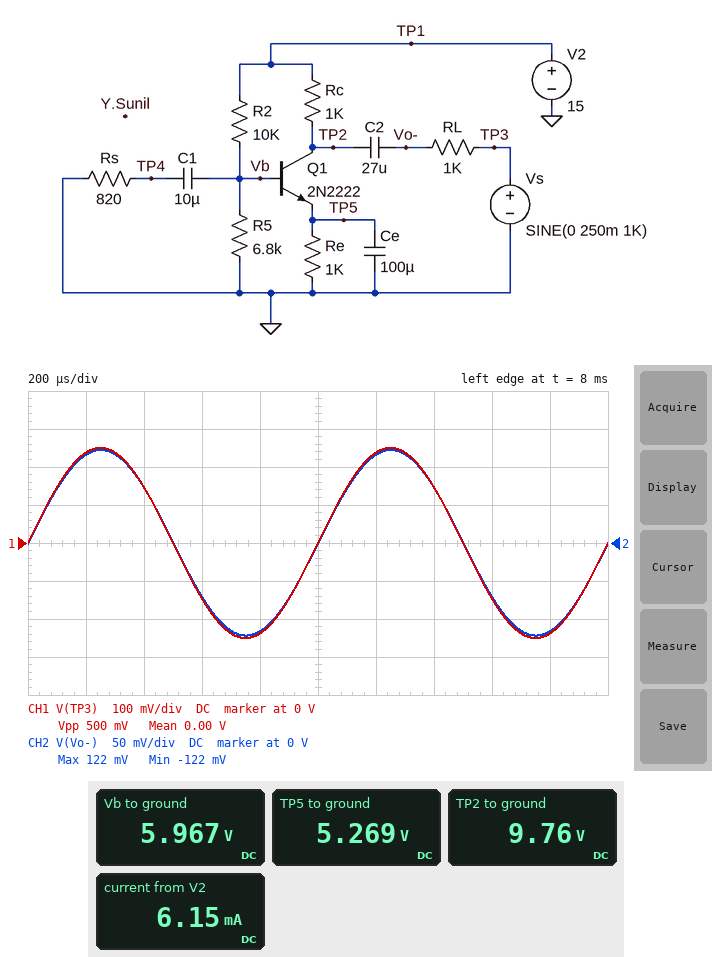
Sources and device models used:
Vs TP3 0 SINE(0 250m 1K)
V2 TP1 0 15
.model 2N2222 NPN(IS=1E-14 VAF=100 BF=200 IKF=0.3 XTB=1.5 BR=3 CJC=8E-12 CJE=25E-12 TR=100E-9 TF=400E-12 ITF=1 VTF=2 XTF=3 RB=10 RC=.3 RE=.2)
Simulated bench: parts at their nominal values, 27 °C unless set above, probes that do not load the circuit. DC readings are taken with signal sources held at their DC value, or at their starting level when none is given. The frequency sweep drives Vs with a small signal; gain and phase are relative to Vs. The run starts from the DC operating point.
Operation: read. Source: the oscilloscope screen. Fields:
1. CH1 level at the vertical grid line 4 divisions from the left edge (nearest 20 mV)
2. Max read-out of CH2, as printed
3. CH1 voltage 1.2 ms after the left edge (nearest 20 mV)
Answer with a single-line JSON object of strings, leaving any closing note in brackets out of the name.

{"CH1 level at the vertical grid line 4 divisions from the left edge": "-240 mV", "Max read-out of CH2, as printed": "122 mV", "CH1 voltage 1.2 ms after the left edge": "240 mV"}
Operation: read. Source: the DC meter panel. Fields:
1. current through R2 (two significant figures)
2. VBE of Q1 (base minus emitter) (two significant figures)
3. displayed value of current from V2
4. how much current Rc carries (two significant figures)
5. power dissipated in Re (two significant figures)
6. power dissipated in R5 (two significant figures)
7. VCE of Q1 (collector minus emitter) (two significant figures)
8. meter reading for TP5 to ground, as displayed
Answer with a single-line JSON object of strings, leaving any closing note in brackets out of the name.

{"current through R2": "900 µA", "VBE of Q1 (base minus emitter)": "700 mV", "displayed value of current from V2": "6.15 mA", "how much current Rc carries": "5.2 mA", "power dissipated in Re": "28 mW", "power dissipated in R5": "5.2 mW", "VCE of Q1 (collector minus emitter)": "4.5 V", "meter reading for TP5 to ground, as displayed": "5.269 V"}
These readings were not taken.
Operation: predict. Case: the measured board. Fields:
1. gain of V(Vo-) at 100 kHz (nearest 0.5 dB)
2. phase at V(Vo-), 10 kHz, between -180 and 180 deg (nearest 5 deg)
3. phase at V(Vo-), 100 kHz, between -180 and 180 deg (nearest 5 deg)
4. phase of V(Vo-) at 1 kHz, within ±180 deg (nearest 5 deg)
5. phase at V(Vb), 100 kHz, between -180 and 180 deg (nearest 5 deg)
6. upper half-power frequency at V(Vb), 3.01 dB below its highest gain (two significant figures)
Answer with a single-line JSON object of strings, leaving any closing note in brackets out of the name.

{"gain of V(Vo-) at 100 kHz": "-6.5 dB", "phase at V(Vo-), 10 kHz, between -180 and 180 deg": "0 deg", "phase at V(Vo-), 100 kHz, between -180 and 180 deg": "-5 deg", "phase of V(Vo-) at 1 kHz, within ±180 deg": "0 deg", "phase at V(Vb), 100 kHz, between -180 and 180 deg": "80 deg", "upper half-power frequency at V(Vb), 3.01 dB below its highest gain": "340 MHz"}
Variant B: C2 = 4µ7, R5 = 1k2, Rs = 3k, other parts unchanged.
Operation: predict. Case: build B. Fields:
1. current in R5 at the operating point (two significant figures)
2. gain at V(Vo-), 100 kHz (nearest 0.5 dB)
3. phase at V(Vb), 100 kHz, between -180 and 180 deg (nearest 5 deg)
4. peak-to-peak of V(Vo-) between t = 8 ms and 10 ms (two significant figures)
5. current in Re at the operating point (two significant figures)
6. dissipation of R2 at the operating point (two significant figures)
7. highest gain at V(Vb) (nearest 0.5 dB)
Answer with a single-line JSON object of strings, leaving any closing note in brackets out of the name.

{"current in R5 at the operating point": "1.3 mA", "gain at V(Vo-), 100 kHz": "-6.0 dB", "phase at V(Vb), 100 kHz, between -180 and 180 deg": "85 deg", "peak-to-peak of V(Vo-) between t = 8 ms and 10 ms": "250 mV", "current in Re at the operating point": "950 µA", "dissipation of R2 at the operating point": "18 mW", "highest gain at V(Vb)": "-37.5 dB"}
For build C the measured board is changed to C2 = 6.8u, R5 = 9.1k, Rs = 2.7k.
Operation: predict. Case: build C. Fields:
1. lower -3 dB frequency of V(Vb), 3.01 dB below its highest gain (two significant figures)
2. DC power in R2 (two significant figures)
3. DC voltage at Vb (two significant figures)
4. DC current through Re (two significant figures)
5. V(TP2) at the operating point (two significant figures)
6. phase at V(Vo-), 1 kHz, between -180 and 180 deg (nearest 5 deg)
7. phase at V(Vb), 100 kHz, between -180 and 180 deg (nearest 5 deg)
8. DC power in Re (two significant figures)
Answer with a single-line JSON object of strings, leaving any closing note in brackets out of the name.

{"lower -3 dB frequency of V(Vb), 3.01 dB below its highest gain": "380 kHz", "DC power in R2": "6.4 mW", "DC voltage at Vb": "7.0 V", "DC current through Re": "6.3 mA", "V(TP2) at the operating point": "8.7 V", "phase at V(Vo-), 1 kHz, between -180 and 180 deg": "0 deg", "phase at V(Vb), 100 kHz, between -180 and 180 deg": "75 deg", "DC power in Re": "40 mW"}
